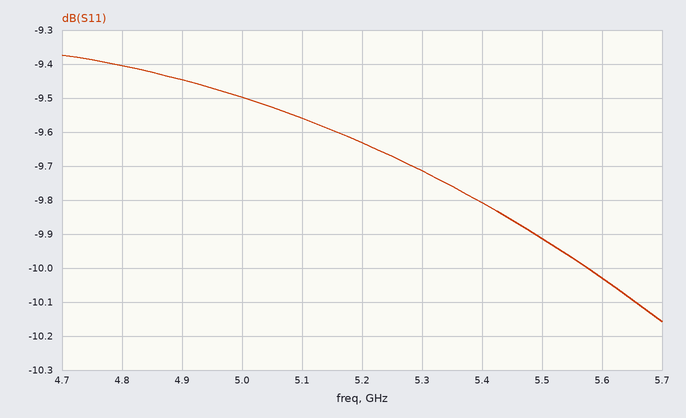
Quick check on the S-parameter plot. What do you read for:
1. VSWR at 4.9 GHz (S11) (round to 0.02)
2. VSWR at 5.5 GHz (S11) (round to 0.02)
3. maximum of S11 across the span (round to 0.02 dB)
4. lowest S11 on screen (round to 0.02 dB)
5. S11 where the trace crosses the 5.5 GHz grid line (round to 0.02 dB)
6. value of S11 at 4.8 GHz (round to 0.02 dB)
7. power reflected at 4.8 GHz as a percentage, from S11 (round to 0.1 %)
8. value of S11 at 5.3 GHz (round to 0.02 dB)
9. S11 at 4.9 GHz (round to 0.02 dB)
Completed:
2.02
1.94
-9.38 dB
-10.16 dB
-9.92 dB
-9.40 dB
11.5 %
-9.72 dB
-9.44 dB
